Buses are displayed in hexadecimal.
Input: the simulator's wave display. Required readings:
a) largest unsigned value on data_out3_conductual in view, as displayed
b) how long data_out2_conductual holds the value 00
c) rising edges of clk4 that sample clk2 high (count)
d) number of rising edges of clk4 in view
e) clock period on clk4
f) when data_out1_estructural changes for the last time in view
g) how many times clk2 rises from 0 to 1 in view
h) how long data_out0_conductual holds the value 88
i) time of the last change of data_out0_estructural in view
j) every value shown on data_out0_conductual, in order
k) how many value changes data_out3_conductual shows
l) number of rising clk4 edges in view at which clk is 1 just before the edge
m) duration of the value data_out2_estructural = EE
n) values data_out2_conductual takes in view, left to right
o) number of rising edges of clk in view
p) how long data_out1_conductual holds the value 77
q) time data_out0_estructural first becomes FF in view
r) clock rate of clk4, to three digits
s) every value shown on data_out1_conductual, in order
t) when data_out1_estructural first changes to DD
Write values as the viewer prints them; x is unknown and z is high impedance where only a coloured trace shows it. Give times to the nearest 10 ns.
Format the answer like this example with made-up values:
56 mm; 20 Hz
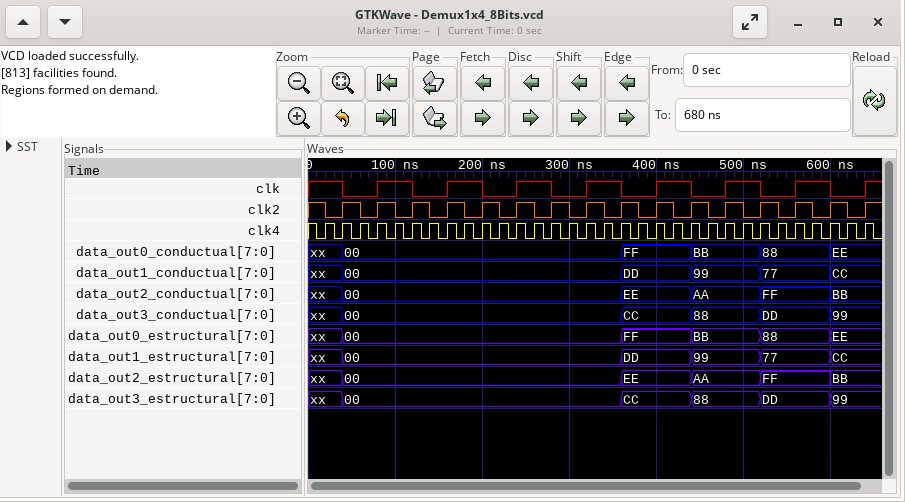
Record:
DD; 320 ns; 16; 32; 20 ns; 600 ns; 16; 80 ns; 600 ns; xx, 00, FF, BB, 88, EE; 5; 16; 80 ns; xx, 00, EE, AA, FF, BB; 8; 80 ns; 360 ns; 50.0 MHz; xx, 00, DD, 99, 77, CC; 360 ns
